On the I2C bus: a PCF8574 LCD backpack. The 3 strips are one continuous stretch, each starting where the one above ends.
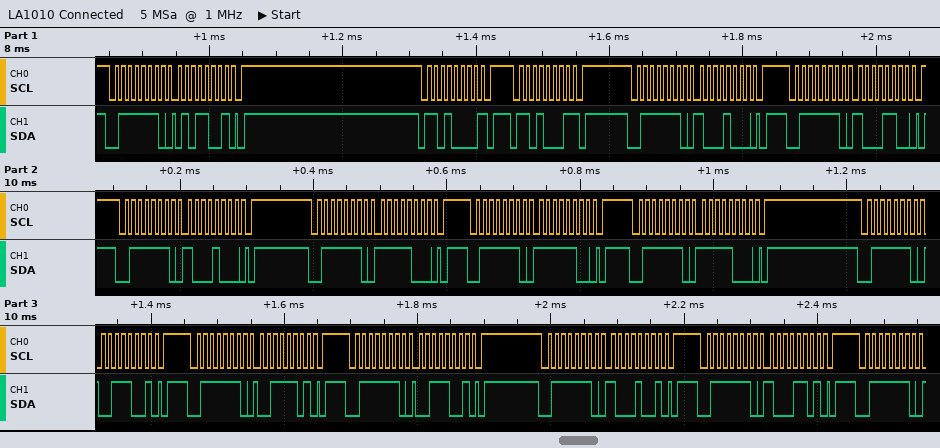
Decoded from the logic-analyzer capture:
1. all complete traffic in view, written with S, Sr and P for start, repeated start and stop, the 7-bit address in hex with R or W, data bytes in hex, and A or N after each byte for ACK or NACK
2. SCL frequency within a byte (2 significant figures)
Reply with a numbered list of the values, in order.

1. S 3FW A 59 A P S 68W N P S 68R N P S 3FW A 88 A P S 3FW A 8C A P S 3FW A 88 A P S 3FW A F8 A P S 3FW A FC A P S 3FW A F8 A P S 3FW A 39 A P S 3FW A 3D A P S 3FW A 39 A P S 3FW A 89 A P S 3FW A 8D A P S 3FW A
2. 100 kHz
